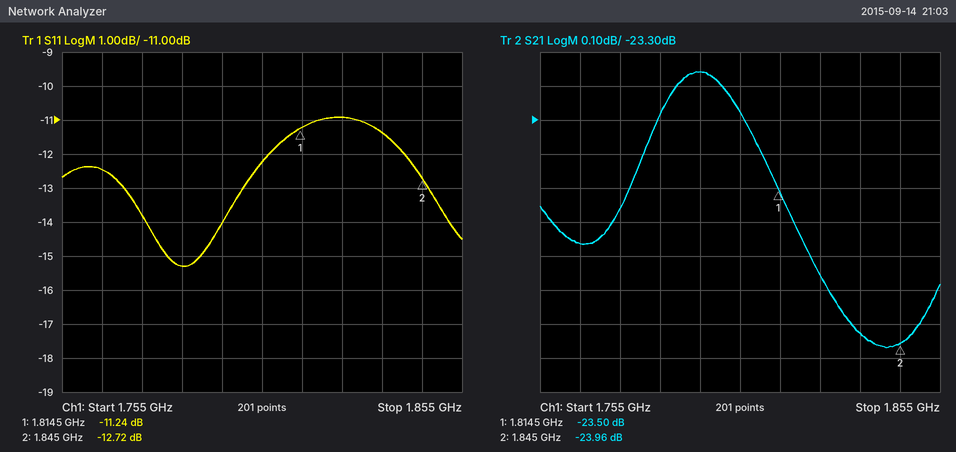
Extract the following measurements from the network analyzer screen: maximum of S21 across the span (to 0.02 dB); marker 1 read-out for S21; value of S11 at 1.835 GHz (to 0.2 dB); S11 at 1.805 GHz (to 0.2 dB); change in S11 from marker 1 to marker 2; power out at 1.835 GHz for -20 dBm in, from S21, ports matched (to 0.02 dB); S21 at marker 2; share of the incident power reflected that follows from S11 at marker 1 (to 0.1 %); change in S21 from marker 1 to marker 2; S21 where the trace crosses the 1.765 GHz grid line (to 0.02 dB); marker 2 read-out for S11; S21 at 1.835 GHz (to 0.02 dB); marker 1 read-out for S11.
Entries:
-23.16 dB
-23.50 dB
-11.4 dB
-12.2 dB
-1.48 dB
-43.92 dBm
-23.96 dB
7.5 %
-0.46 dB
-23.66 dB
-12.72 dB
-23.92 dB
-11.24 dB
